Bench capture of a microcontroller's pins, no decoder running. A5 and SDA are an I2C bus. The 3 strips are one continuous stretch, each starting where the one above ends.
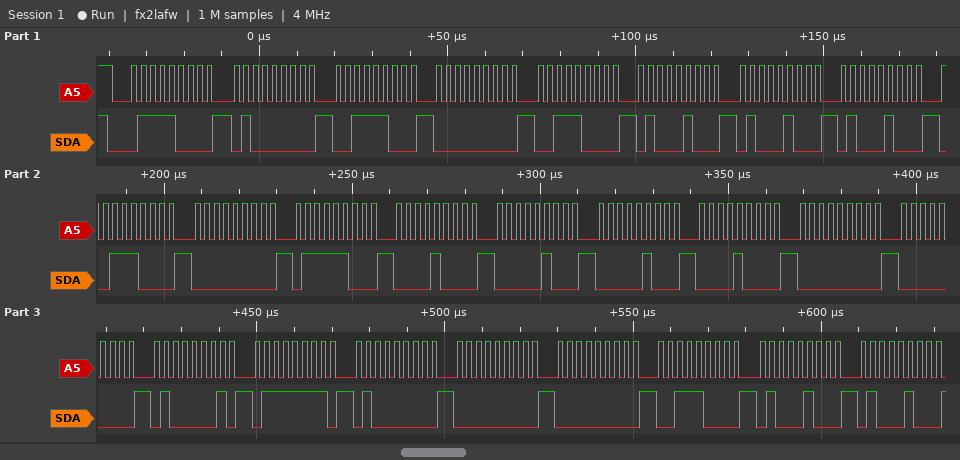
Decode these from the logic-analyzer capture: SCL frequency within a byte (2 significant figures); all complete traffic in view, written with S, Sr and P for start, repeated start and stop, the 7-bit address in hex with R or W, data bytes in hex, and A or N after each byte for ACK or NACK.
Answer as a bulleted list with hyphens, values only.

- 400 kHz
- S 3CW A 40 A 3C A 00 A 38 A 44 A 44 A 44 A 38 A 00 A 7C A 08 A 04 A 04 A 08 A 00 A 00 A 41 A 7F A 40 A 00 A 00 A 38 A 44 A 44 A
